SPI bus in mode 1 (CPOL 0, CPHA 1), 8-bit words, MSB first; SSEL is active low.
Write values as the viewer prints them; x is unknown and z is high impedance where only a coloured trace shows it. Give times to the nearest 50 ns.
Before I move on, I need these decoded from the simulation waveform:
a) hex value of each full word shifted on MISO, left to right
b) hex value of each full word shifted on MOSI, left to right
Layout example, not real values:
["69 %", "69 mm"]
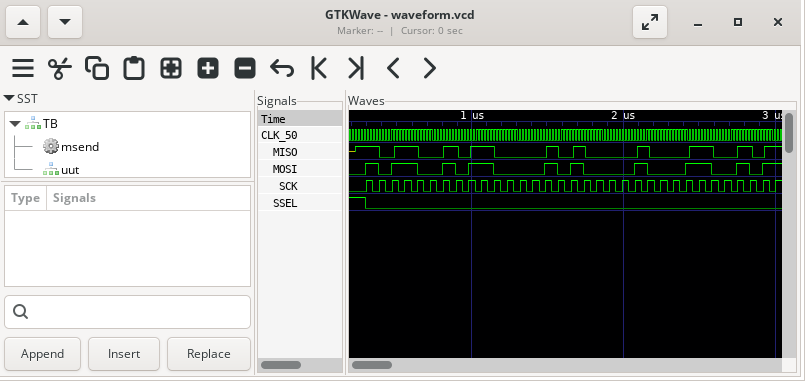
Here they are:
["B2, C2, 84, 65", "B2, C2, 84, 65"]
